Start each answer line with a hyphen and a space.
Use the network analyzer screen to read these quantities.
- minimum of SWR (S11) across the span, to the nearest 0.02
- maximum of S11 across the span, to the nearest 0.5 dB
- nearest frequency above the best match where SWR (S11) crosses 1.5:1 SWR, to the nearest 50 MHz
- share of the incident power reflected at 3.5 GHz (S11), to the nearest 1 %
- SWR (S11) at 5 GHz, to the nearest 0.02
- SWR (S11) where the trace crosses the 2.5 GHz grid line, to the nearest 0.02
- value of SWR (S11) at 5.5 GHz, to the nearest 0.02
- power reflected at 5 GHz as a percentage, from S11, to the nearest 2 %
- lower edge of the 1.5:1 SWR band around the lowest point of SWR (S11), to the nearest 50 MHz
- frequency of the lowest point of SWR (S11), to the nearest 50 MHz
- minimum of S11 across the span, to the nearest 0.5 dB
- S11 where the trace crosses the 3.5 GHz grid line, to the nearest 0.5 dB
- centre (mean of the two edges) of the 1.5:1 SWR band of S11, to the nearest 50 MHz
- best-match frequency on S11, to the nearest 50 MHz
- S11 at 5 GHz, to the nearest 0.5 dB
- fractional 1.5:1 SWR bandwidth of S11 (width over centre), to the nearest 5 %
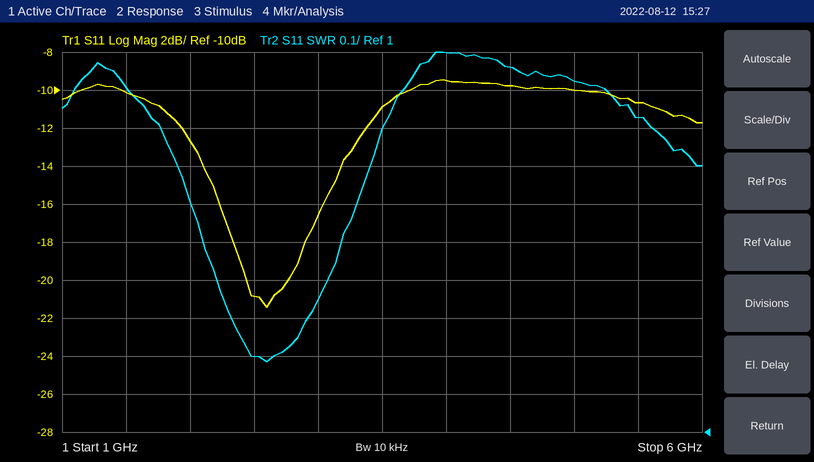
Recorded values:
- 1.18
- -9.5 dB
- 3.20 GHz
- 8 %
- 1.92
- 1.20
- 1.82
- 10 %
- 2.10 GHz
- 2.60 GHz
- -21.5 dB
- -11.0 dB
- 2.65 GHz
- 2.60 GHz
- -10.0 dB
- 40 %
